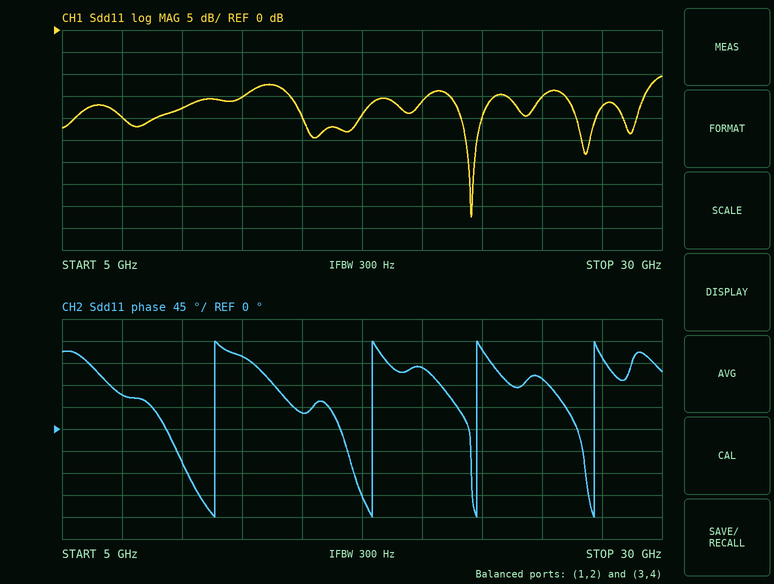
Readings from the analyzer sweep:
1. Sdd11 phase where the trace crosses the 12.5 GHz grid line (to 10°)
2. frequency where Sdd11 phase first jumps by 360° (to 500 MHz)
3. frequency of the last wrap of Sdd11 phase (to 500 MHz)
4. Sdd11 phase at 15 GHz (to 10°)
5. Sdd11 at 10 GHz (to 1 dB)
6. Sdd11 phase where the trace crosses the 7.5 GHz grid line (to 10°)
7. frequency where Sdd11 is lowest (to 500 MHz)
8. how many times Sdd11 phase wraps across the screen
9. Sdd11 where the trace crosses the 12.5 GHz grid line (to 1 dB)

150°
11.5 GHz
27.0 GHz
30°
-18 dB
70°
22.0 GHz
4
-15 dB
